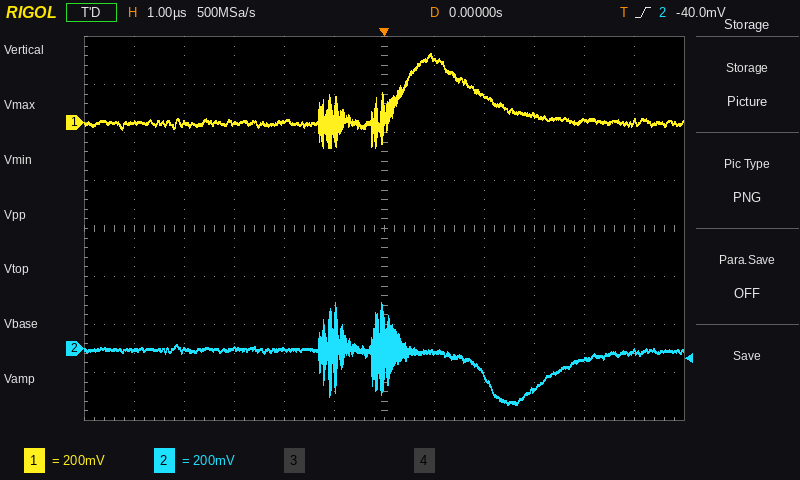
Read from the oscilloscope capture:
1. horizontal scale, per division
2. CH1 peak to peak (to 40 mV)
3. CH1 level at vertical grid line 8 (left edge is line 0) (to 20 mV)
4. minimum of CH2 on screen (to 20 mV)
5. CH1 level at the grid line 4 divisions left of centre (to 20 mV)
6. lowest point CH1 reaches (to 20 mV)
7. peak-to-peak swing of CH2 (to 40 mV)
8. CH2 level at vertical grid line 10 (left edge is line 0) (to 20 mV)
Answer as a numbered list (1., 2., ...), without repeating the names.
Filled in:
1. 1 µs
2. 400 mV
3. 120 mV
4. -240 mV
5. 0 mV
6. -100 mV
7. 440 mV
8. -40 mV
